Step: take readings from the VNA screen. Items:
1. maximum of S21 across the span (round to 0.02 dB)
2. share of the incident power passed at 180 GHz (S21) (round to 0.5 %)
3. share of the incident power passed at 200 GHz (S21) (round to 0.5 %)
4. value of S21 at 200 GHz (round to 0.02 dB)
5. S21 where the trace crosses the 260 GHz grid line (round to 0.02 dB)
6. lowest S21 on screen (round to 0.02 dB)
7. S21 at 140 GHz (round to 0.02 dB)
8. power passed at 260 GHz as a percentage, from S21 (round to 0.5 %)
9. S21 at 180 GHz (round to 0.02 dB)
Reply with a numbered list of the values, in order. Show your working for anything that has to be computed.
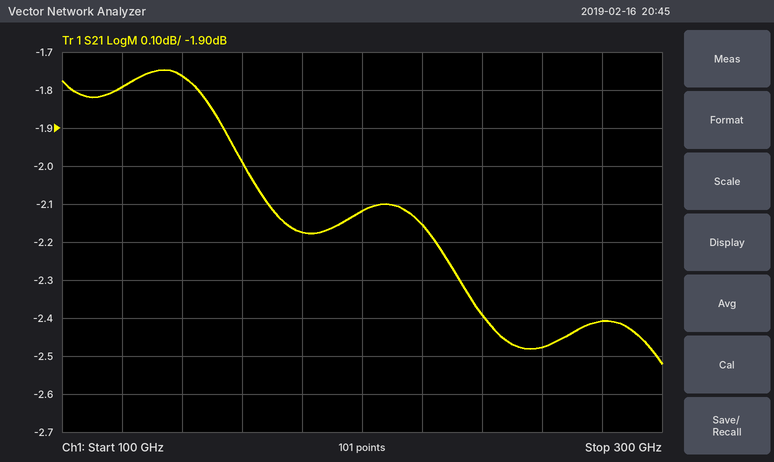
1. -1.74 dB
2. 10^(-2.18/10) ≈ 60.5 %
3. 10^(-2.12/10) ≈ 61.4 %, so 61.5 % to the nearest 0.5 %
4. -2.12 dB
5. -2.48 dB
6. -2.52 dB
7. -1.76 dB
8. 10^(-2.48/10) ≈ 56.5 %
9. -2.18 dB
